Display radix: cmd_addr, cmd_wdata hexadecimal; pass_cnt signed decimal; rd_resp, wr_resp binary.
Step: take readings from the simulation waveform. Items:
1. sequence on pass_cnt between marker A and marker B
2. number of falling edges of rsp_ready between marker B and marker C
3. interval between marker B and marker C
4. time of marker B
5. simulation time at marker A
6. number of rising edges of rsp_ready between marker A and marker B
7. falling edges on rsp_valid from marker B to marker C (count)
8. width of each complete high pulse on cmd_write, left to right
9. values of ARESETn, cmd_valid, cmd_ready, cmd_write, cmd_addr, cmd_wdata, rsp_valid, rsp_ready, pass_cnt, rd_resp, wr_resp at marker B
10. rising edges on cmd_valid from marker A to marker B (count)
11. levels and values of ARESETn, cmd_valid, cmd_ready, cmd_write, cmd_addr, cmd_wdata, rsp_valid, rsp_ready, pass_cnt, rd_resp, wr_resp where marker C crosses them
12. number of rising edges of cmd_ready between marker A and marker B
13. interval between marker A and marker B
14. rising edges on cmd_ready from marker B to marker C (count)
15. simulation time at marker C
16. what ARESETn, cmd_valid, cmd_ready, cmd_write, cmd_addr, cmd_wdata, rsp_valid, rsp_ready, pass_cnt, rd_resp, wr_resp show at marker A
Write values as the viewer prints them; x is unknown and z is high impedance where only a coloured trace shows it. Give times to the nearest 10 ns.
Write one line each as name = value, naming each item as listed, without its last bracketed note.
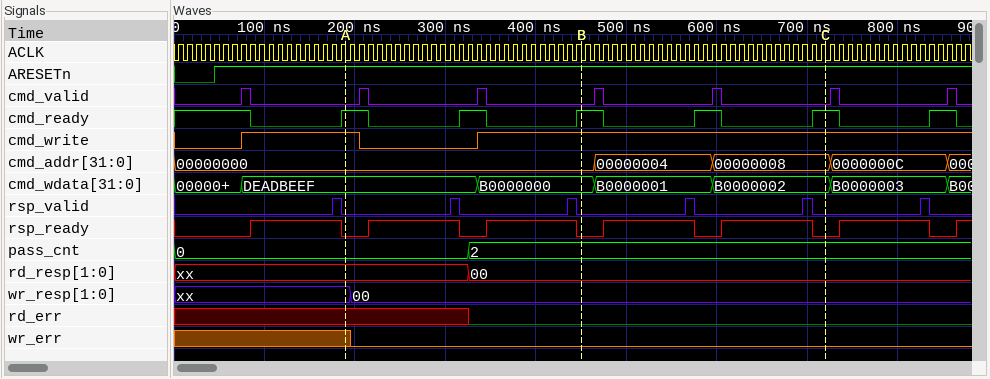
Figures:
sequence on pass_cnt between marker A and marker B = 0, 2
number of falling edges of rsp_ready between marker B and marker C = 2
interval between marker B and marker C = 270 ns
time of marker B = 450 ns
simulation time at marker A = 190 ns
number of rising edges of rsp_ready between marker A and marker B = 2
falling edges on rsp_valid from marker B to marker C = 2
width of each complete high pulse on cmd_write, left to right = 130 ns
values of ARESETn, cmd_valid, cmd_ready, cmd_write, cmd_addr, cmd_wdata, rsp_valid, rsp_ready, pass_cnt, rd_resp, wr_resp at marker B = ARESETn=1, cmd_valid=0, cmd_ready=1, cmd_write=1, cmd_addr=00000000, cmd_wdata=B0000000, rsp_valid=0, rsp_ready=0, pass_cnt=2, rd_resp=00, wr_resp=00
rising edges on cmd_valid from marker A to marker B = 2
levels and values of ARESETn, cmd_valid, cmd_ready, cmd_write, cmd_addr, cmd_wdata, rsp_valid, rsp_ready, pass_cnt, rd_resp, wr_resp where marker C crosses them = ARESETn=1, cmd_valid=0, cmd_ready=1, cmd_write=1, cmd_addr=00000008, cmd_wdata=B0000002, rsp_valid=0, rsp_ready=0, pass_cnt=2, rd_resp=00, wr_resp=00
number of rising edges of cmd_ready between marker A and marker B = 2
interval between marker A and marker B = 260 ns
rising edges on cmd_ready from marker B to marker C = 2
simulation time at marker C = 720 ns
what ARESETn, cmd_valid, cmd_ready, cmd_write, cmd_addr, cmd_wdata, rsp_valid, rsp_ready, pass_cnt, rd_resp, wr_resp show at marker A = ARESETn=1, cmd_valid=0, cmd_ready=1, cmd_write=1, cmd_addr=00000000, cmd_wdata=DEADBEEF, rsp_valid=0, rsp_ready=0, pass_cnt=0, rd_resp=xx, wr_resp=xx
